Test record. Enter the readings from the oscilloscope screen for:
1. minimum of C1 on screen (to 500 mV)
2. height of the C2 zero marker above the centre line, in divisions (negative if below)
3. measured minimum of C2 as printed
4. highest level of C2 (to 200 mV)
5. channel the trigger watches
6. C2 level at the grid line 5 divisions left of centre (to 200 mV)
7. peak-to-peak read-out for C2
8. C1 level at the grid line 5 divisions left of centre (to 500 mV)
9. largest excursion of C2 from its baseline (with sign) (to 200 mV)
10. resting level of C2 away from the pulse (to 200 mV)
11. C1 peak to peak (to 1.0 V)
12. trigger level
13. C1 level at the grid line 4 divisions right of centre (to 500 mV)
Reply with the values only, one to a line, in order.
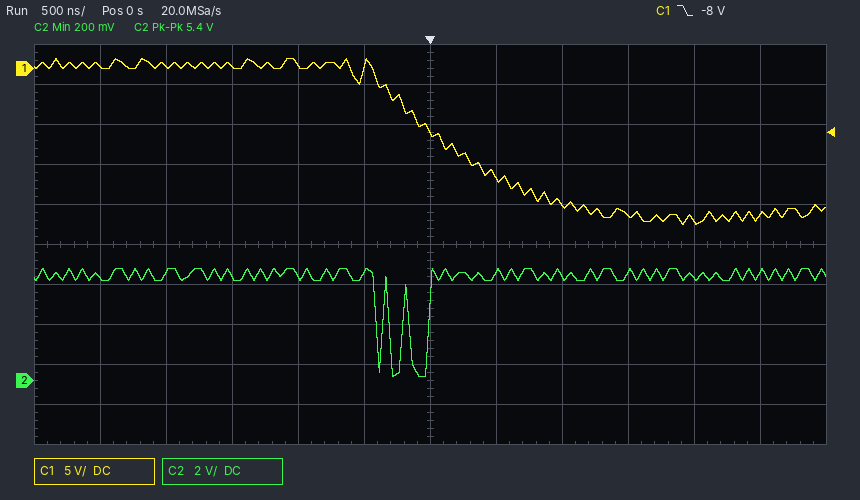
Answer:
-19.5 V
-3.4 div
200 mV
5.6 V
C1
5.2 V
5.4 V
500 mV
-5.0 V
5.2 V
21.0 V
-8 V
-19.0 V
